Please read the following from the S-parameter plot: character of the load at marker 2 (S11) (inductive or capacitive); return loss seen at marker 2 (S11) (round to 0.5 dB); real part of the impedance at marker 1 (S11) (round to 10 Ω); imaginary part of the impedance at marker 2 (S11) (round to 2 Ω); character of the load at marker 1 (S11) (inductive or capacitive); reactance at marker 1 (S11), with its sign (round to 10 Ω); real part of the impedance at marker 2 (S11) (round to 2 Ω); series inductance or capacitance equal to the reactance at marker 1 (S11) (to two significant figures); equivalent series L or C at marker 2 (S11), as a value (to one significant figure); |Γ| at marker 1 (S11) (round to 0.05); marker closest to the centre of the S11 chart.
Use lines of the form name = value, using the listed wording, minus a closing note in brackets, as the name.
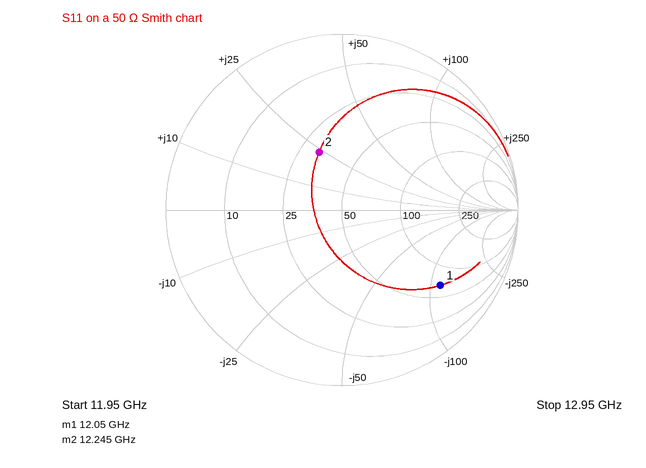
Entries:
character of the load at marker 2 (S11) = inductive
return loss seen at marker 2 (S11) = 9.0 dB
real part of the impedance at marker 1 (S11) = 70 Ω
imaginary part of the impedance at marker 2 (S11) = +24 Ω
character of the load at marker 1 (S11) = capacitive
reactance at marker 1 (S11), with its sign = -110 Ω
real part of the impedance at marker 2 (S11) = 32 Ω
series inductance or capacitance equal to the reactance at marker 1 (S11) = 120 fF
equivalent series L or C at marker 2 (S11), as a value = 300 pH
|Γ| at marker 1 (S11) = 0.70
marker closest to the centre of the S11 chart = marker 2
